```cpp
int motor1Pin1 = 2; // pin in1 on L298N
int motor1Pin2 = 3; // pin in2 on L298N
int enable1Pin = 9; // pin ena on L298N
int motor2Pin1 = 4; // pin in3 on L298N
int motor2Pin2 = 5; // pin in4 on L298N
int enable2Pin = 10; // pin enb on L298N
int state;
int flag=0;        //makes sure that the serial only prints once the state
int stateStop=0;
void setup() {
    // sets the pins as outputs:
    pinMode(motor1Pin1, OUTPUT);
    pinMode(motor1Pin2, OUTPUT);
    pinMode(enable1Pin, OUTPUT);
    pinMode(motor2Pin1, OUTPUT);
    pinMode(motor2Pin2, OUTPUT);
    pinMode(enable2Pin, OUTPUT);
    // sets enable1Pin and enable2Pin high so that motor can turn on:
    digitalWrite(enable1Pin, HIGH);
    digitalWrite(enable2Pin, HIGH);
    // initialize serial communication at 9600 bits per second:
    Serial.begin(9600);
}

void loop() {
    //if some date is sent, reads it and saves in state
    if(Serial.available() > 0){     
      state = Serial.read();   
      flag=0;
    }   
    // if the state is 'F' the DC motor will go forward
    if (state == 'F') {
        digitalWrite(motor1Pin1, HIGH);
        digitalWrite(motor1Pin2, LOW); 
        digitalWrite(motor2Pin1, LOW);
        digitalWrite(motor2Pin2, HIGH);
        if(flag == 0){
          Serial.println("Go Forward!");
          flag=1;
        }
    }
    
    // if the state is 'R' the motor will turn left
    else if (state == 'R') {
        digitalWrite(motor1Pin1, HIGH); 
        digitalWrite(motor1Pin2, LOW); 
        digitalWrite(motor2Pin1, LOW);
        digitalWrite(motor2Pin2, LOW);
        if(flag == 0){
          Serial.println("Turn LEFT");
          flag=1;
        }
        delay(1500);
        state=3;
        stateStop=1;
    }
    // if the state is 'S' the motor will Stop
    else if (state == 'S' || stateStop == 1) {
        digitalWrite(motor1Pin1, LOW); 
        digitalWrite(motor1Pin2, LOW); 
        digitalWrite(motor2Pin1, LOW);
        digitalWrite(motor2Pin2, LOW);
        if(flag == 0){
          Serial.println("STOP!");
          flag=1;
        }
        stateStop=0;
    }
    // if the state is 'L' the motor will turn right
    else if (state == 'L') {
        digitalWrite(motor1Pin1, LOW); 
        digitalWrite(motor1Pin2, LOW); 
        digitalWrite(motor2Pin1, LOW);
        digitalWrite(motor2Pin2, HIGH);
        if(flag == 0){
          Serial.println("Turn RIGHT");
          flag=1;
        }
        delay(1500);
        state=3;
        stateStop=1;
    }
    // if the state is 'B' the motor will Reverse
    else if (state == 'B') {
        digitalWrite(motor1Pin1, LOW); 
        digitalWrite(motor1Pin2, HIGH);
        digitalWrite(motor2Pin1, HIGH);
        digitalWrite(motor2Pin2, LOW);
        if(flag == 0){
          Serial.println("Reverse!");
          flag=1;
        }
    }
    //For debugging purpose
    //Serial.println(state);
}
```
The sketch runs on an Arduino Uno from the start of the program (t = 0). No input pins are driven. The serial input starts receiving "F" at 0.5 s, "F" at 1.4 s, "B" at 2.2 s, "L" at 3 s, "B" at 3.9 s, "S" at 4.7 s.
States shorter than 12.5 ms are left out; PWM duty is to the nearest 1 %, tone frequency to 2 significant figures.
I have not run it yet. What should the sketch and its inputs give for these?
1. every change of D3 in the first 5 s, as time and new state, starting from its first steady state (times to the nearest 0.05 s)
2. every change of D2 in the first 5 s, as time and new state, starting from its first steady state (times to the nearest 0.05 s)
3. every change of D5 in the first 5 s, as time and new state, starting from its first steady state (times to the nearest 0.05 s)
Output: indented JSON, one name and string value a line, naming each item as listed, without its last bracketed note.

{
  "every change of D3 in the first 5 s, as time and new state, starting from its first steady state": "0 s low; 2.2 s high; 3 s low; 4.5 s high; 4.7 s low",
  "every change of D2 in the first 5 s, as time and new state, starting from its first steady state": "0 s low; 0.5 s high; 2.2 s low",
  "every change of D5 in the first 5 s, as time and new state, starting from its first steady state": "0 s low; 0.5 s high; 2.2 s low; 3 s high; 4.5 s low"
}
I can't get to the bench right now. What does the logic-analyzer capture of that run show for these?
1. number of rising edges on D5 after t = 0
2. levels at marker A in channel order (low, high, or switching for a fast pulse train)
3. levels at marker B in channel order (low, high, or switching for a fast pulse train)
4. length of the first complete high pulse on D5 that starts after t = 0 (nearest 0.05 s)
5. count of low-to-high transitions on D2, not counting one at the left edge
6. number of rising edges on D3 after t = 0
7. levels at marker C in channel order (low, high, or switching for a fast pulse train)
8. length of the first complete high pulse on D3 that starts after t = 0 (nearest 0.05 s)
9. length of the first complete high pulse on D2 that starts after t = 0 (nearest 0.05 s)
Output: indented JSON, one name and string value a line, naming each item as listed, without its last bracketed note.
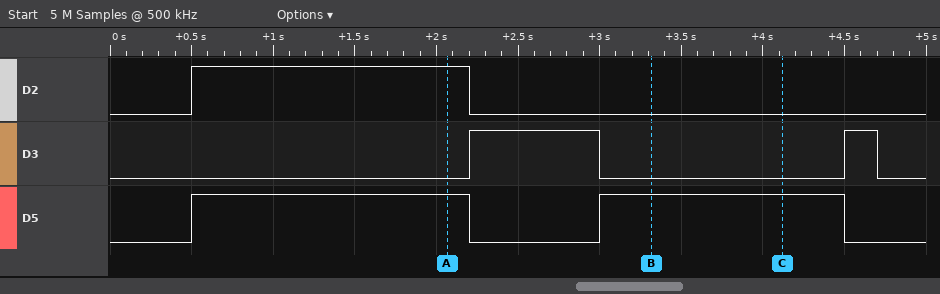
{
  "number of rising edges on D5 after t = 0": "2",
  "levels at marker A in channel order": "D2 high, D3 low, D5 high",
  "levels at marker B in channel order": "D2 low, D3 low, D5 high",
  "length of the first complete high pulse on D5 that starts after t = 0": "1.70 s",
  "count of low-to-high transitions on D2, not counting one at the left edge": "1",
  "number of rising edges on D3 after t = 0": "2",
  "levels at marker C in channel order": "D2 low, D3 low, D5 high",
  "length of the first complete high pulse on D3 that starts after t = 0": "0.80 s",
  "length of the first complete high pulse on D2 that starts after t = 0": "1.70 s"
}
